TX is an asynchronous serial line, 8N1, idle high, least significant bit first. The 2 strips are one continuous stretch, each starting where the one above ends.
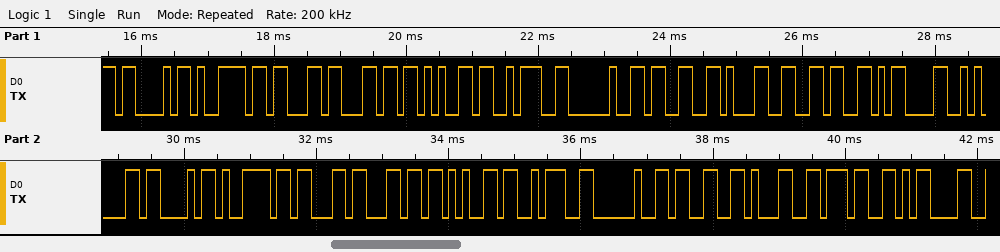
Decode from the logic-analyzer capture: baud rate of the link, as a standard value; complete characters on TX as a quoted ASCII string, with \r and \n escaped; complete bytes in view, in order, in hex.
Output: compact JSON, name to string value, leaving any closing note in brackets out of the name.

{"baud rate of the link, as a standard value": "9600 baud", "complete characters on TX as a quoted ASCII string, with \\r and \\n escaped": "\"Cycle: 316\\r\\nCycle: 317\\r\"", "complete bytes in view, in order, in hex": "43 79 63 6C 65 3A 20 33 31 36 0D 0A 43 79 63 6C 65 3A 20 33 31 37 0D"}
